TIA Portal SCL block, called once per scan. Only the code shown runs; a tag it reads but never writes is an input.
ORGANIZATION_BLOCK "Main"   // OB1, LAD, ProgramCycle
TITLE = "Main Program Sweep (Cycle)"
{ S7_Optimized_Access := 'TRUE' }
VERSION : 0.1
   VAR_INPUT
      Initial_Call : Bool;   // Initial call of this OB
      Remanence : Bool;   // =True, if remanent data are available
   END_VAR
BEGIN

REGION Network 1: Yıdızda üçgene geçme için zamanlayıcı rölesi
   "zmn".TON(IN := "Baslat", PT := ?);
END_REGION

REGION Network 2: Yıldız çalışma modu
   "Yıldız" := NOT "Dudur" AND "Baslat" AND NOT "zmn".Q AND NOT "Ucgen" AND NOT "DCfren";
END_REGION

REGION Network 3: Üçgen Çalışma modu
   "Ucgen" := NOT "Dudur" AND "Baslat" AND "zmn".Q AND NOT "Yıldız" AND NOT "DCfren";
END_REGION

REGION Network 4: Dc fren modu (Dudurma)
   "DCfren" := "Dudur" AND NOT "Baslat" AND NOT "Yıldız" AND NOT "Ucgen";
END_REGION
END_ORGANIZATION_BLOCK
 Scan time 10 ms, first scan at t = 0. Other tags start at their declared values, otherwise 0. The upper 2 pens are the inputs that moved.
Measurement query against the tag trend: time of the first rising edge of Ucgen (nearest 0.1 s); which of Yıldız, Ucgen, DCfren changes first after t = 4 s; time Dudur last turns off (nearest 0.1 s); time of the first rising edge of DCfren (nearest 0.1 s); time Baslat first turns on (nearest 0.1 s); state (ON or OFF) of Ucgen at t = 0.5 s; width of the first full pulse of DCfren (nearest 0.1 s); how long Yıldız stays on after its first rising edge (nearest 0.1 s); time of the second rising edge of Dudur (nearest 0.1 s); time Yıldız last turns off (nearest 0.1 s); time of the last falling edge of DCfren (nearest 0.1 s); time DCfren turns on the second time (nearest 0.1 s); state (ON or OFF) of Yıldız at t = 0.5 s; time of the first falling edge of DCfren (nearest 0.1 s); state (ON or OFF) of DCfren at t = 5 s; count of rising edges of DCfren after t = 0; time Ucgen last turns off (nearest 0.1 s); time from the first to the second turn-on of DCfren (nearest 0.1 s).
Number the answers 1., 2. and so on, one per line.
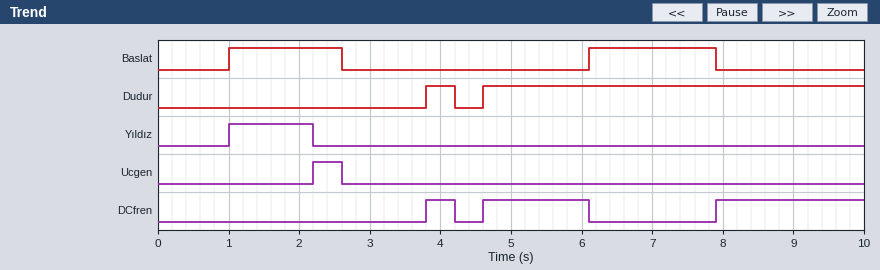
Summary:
1. 2.2 s
2. DCfren
3. 4.2 s
4. 3.8 s
5. 1.0 s
6. OFF
7. 0.4 s
8. 1.2 s
9. 4.6 s
10. 2.2 s
11. 6.1 s
12. 4.6 s
13. OFF
14. 4.2 s
15. ON
16. 3
17. 2.6 s
18. 0.8 s
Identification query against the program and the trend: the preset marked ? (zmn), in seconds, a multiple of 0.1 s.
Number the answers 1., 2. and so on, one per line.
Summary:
1. 1.2 s
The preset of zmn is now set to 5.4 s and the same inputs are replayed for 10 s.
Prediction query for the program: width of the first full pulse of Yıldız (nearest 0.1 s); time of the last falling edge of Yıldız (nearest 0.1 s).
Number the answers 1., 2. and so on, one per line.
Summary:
1. 1.6 s
2. 2.6 s
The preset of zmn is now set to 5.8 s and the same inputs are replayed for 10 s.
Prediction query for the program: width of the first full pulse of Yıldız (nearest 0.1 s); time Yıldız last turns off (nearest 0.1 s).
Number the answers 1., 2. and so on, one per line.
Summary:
1. 1.6 s
2. 2.6 s
